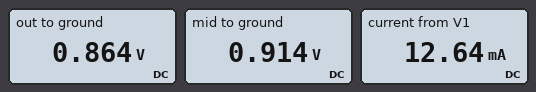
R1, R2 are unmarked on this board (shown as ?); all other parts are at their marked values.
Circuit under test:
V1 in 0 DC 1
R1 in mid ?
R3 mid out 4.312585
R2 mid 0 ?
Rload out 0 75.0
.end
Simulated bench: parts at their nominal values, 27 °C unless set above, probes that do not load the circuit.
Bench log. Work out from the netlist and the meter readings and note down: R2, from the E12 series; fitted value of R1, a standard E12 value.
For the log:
820 Ω
6.8 Ω
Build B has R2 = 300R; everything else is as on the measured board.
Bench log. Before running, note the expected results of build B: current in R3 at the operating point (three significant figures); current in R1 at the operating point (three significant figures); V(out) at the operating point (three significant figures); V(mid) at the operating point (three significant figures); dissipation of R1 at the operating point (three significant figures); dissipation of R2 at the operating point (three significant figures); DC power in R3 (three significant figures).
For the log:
11.4 mA
14.4 mA
853 mV
902 mV
1.41 mW
2.71 mW
558 µW
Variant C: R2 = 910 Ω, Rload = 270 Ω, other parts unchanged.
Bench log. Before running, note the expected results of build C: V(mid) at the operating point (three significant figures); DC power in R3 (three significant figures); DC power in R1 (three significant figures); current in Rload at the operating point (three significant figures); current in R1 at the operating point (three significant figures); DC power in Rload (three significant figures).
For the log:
969 mV
53.8 µW
144 µW
3.53 mA
4.60 mA
3.37 mW
